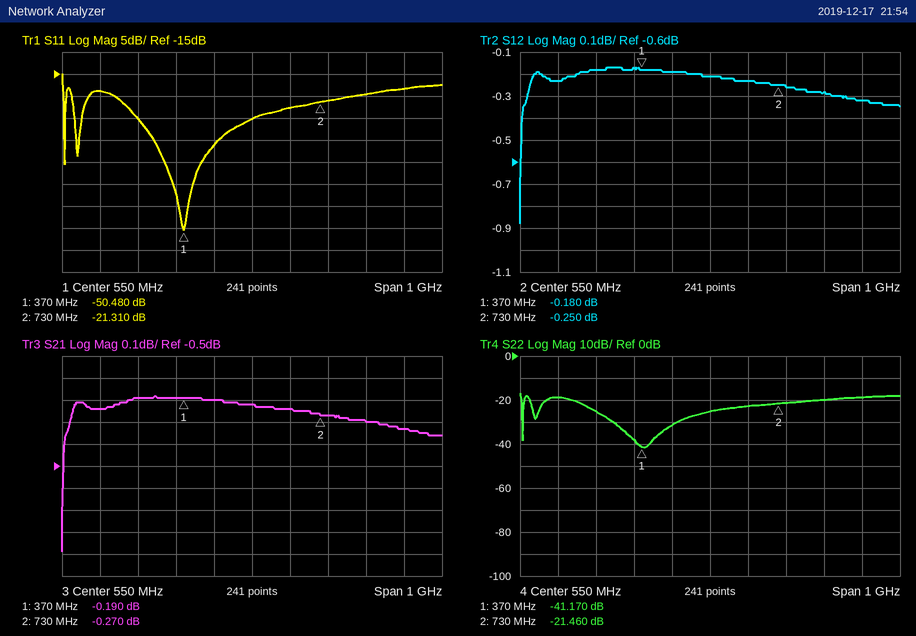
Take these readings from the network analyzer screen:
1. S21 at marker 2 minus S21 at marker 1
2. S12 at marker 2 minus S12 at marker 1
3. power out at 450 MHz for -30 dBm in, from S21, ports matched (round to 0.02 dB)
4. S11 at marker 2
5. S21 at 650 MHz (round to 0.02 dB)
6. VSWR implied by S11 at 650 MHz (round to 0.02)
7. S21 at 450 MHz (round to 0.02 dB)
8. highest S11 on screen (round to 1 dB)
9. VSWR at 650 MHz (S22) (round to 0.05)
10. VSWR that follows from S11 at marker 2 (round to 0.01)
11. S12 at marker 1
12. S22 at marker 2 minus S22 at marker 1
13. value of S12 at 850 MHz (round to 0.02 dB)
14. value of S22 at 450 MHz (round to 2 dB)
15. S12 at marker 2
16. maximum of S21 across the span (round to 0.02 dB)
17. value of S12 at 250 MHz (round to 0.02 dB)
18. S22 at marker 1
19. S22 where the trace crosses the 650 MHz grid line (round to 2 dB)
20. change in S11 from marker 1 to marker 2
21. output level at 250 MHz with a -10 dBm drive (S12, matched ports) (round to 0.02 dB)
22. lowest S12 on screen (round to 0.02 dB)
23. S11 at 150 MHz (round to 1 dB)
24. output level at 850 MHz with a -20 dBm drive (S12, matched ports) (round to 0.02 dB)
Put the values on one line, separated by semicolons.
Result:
-0.080 dB; -0.070 dB; -30.20 dBm; -21.310 dB; -0.24 dB; 1.16; -0.20 dB; -15 dB; 1.15; 1.19; -0.180 dB; 19.710 dB; -0.28 dB; -32 dB; -0.250 dB; -0.18 dB; -0.18 dB; -41.170 dB; -22 dB; 29.170 dB; -10.18 dBm; -0.88 dB; -19 dB; -20.28 dBm
